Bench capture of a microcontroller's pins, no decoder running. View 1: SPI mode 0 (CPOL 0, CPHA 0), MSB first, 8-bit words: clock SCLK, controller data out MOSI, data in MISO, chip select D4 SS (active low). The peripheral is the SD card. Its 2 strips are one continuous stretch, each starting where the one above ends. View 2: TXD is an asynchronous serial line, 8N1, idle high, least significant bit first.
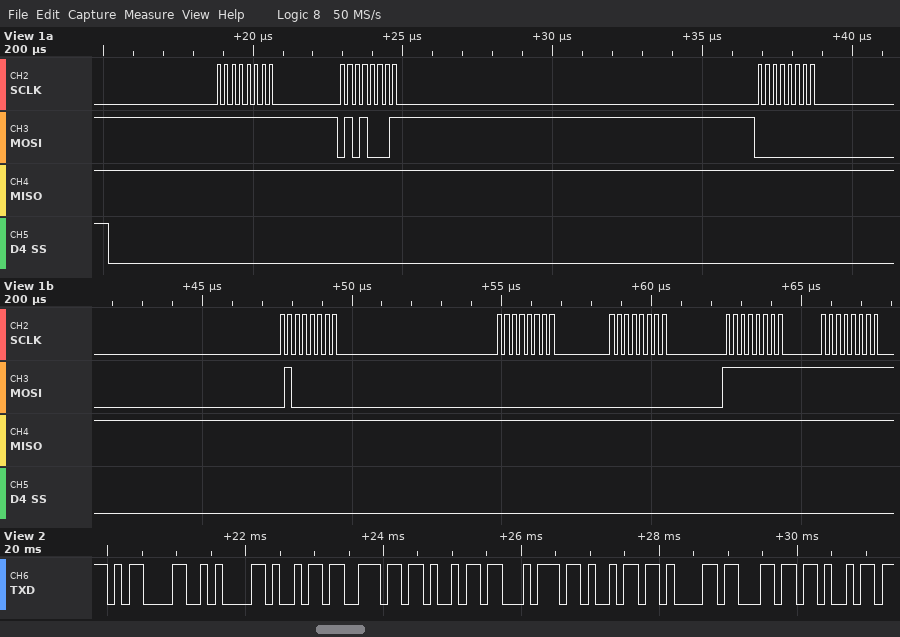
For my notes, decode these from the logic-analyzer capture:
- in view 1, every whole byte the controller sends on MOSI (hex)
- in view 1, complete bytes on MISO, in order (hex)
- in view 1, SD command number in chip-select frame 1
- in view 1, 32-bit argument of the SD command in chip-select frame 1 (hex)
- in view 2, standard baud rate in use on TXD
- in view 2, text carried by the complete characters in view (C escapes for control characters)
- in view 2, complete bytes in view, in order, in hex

0xFF 0x51 0x00 0x40 0x00 0x00 0xFF 0xFF
0xFF 0xFF 0xFF 0xFF 0xFF 0xFF 0xFF 0xFF
CMD17
0x00400000
9600 baud
"\r\ninitiali"
0D 0A 69 6E 69 74 69 61 6C 69
